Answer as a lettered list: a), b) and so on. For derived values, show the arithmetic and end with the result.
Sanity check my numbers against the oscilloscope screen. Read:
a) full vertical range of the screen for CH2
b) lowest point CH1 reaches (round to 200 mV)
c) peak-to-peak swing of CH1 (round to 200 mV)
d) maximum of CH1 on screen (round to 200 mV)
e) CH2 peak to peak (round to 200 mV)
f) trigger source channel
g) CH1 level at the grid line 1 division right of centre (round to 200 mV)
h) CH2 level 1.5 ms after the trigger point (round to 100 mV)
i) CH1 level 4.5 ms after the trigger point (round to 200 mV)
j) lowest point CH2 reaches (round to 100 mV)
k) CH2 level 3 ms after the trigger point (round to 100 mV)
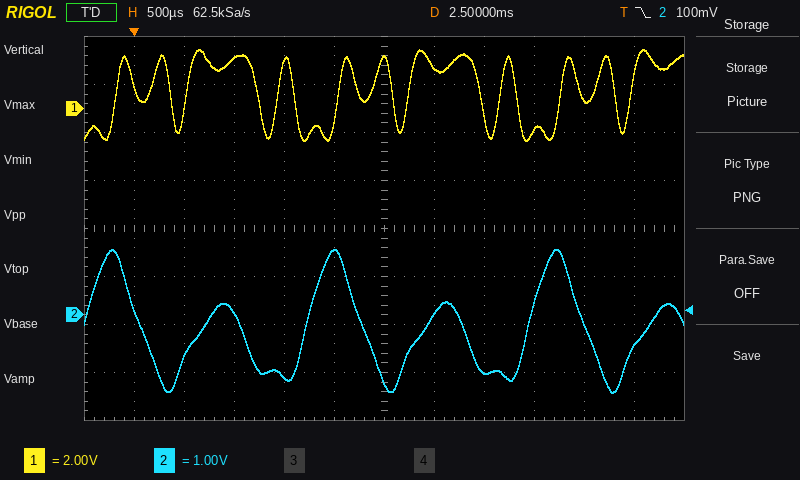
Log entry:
a) 8 V
b) -1.4 V
c) 2.4 V − (-1.4 V) = 3.8 V
d) 2.4 V
e) 3.0 V
f) CH2
g) 1.8 V
h) -1.3 V
i) 400 mV
j) -1.6 V
k) 0.0 V
